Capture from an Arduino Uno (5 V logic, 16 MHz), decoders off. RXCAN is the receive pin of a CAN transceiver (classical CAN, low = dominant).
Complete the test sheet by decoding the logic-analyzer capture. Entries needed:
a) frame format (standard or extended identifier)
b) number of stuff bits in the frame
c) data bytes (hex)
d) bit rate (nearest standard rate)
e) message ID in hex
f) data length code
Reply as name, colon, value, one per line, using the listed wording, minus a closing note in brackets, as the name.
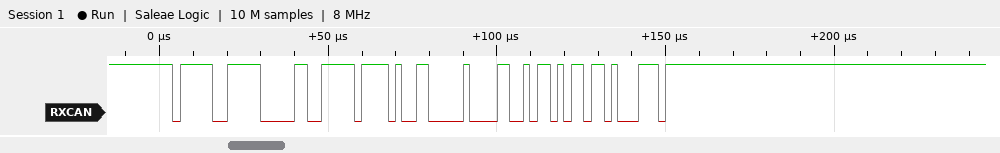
frame format: standard
number of stuff bits in the frame: 5
data bytes: FF A6 00 CB
bit rate: 500 kbit/s
message ID in hex: 0x7DF
data length code: 4
